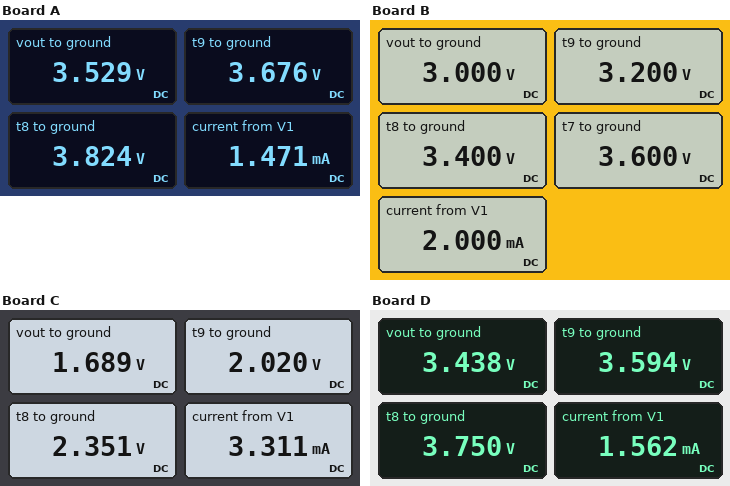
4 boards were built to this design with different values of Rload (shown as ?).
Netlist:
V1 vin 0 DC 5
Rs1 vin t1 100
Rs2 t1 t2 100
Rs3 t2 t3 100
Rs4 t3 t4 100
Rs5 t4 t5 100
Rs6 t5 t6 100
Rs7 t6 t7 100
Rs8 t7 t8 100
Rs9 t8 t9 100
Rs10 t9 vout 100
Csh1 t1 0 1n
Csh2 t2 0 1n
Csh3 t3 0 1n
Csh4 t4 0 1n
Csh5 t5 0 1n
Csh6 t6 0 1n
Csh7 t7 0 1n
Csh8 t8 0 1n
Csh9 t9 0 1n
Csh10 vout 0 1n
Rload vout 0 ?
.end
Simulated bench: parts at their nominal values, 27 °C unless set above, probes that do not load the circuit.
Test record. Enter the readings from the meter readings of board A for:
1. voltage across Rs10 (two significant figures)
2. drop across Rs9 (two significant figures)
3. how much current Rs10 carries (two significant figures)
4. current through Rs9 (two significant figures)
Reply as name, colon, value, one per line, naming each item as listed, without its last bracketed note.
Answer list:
voltage across Rs10: 150 mV
drop across Rs9: 150 mV
how much current Rs10 carries: 1.5 mA
current through Rs9: 1.5 mA
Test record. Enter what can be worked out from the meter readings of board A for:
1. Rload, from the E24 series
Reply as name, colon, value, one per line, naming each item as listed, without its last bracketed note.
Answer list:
Rload, from the E24 series: 2.4 kΩ
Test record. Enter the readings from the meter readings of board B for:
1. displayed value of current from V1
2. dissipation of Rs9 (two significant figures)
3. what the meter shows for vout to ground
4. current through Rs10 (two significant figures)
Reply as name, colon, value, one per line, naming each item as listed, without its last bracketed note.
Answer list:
displayed value of current from V1: 2.000 mA
dissipation of Rs9: 400 µW
what the meter shows for vout to ground: 3.000 V
current through Rs10: 2.0 mA
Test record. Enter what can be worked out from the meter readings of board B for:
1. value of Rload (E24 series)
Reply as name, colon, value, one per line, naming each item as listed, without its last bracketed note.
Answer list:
value of Rload: 1.5 kΩ
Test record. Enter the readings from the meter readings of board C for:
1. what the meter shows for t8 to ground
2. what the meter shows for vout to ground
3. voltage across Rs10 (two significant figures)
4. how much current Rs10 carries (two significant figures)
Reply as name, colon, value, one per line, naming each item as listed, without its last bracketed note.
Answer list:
what the meter shows for t8 to ground: 2.351 V
what the meter shows for vout to ground: 1.689 V
voltage across Rs10: 330 mV
how much current Rs10 carries: 3.3 mA
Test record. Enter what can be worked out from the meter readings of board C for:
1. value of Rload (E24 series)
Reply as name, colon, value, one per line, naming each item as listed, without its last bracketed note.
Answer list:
value of Rload: 510 Ω
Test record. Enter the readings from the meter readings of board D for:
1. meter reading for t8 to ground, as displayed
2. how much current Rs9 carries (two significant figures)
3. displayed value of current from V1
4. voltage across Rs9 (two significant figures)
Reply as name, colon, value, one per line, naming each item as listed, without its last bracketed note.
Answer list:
meter reading for t8 to ground, as displayed: 3.750 V
how much current Rs9 carries: 1.6 mA
displayed value of current from V1: 1.562 mA
voltage across Rs9: 160 mV
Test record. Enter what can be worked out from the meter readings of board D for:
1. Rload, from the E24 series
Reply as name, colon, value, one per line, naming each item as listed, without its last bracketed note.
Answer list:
Rload, from the E24 series: 2.2 kΩ
